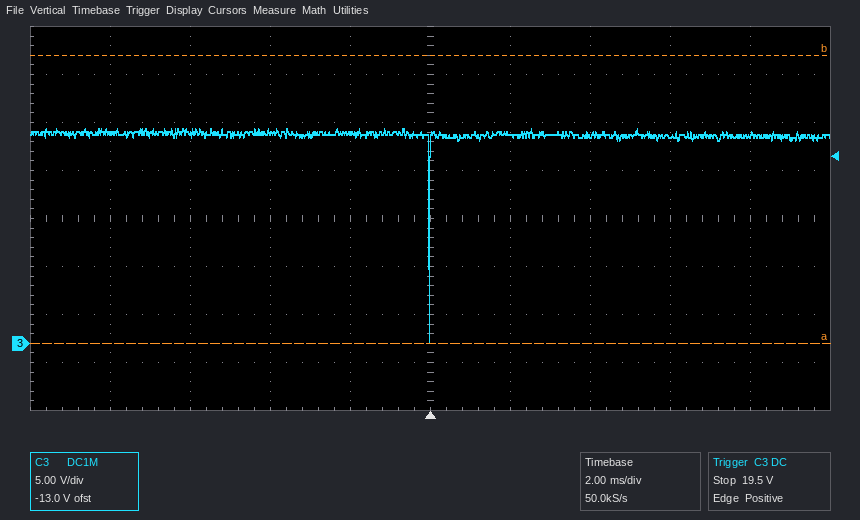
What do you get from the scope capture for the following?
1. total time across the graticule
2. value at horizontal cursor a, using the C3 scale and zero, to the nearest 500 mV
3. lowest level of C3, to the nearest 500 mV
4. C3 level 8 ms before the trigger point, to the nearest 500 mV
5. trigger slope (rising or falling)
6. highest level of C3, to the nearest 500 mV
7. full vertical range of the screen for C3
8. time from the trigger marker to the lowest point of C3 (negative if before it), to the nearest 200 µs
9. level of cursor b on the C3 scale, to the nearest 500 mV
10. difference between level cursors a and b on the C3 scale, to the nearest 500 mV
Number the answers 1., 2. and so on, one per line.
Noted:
1. 20 ms
2. 0.0 V
3. 0.0 V
4. 22.0 V
5. rising
6. 22.5 V
7. 40 V
8. 0.0 ms
9. 30.0 V
10. 30.0 V
